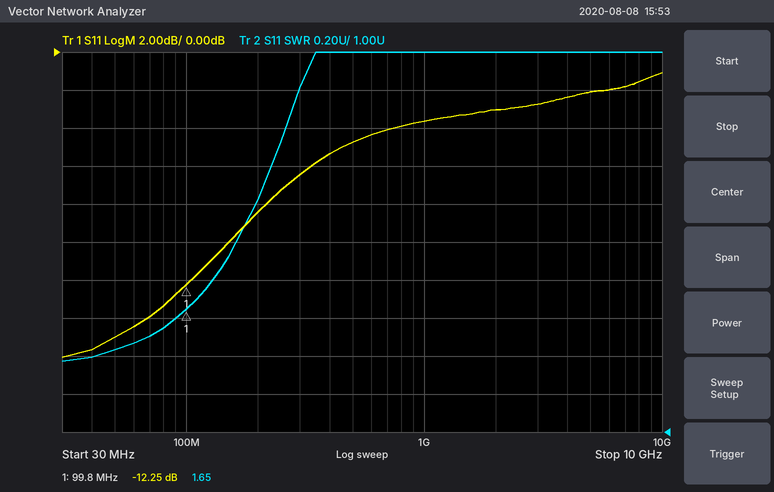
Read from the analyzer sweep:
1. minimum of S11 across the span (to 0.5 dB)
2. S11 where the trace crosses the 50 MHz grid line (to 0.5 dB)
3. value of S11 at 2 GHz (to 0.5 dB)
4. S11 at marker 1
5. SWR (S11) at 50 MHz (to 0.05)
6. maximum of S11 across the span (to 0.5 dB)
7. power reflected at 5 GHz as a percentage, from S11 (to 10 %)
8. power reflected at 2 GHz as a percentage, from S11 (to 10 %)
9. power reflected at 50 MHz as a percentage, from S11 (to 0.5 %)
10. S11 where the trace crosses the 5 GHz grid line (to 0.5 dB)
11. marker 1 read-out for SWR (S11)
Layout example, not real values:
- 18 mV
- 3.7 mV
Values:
- -16.0 dB
- -15.0 dB
- -3.0 dB
- -12.25 dB
- 1.45
- -1.0 dB
- 60 %
- 50 %
- 3.0 %
- -2.0 dB
- 1.65
